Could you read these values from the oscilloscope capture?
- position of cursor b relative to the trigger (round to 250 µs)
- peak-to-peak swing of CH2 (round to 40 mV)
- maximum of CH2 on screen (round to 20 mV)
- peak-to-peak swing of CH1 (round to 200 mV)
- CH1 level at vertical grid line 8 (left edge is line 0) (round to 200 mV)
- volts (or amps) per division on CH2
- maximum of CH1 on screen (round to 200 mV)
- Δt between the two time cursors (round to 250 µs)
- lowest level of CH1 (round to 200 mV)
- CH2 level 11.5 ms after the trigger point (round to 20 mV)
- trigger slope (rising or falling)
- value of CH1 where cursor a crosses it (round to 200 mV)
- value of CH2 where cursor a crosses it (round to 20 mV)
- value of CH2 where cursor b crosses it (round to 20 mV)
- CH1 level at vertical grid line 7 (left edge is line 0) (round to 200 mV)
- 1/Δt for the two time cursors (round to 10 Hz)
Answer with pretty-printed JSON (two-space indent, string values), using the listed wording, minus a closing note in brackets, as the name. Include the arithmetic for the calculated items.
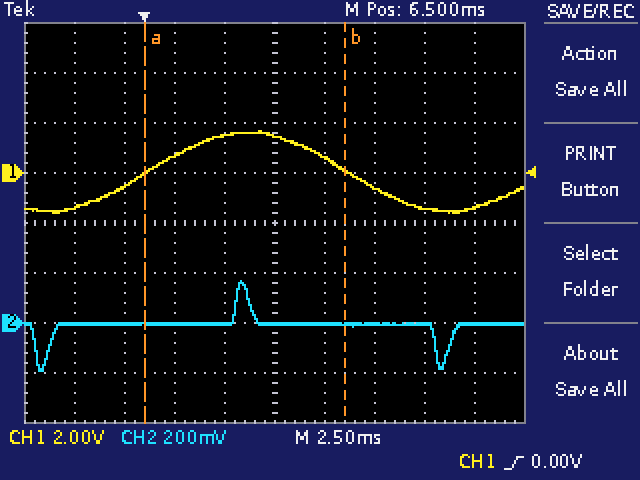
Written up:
{
  "position of cursor b relative to the trigger": "+10.00 ms",
  "peak-to-peak swing of CH2": "360 mV",
  "maximum of CH2 on screen": "160 mV",
  "peak-to-peak swing of CH1": "1.6 V − (-1.6 V) = 3.2 V",
  "CH1 level at vertical grid line 8 (left edge is line 0)": "-1.4 V",
  "volts (or amps) per division on CH2": "200 mV",
  "maximum of CH1 on screen": "1.6 V",
  "Δt between the two time cursors": "10.00 ms",
  "lowest level of CH1": "-1.6 V",
  "CH2 level 11.5 ms after the trigger point": "0 mV",
  "trigger slope": "rising",
  "value of CH1 where cursor a crosses it": "0.0 V",
  "value of CH2 where cursor a crosses it": "0 mV",
  "value of CH2 where cursor b crosses it": "0 mV",
  "CH1 level at vertical grid line 7 (left edge is line 0)": "-600 mV",
  "1/Δt for the two time cursors": "1 / 10.00 ms ≈ 100 Hz"
}
